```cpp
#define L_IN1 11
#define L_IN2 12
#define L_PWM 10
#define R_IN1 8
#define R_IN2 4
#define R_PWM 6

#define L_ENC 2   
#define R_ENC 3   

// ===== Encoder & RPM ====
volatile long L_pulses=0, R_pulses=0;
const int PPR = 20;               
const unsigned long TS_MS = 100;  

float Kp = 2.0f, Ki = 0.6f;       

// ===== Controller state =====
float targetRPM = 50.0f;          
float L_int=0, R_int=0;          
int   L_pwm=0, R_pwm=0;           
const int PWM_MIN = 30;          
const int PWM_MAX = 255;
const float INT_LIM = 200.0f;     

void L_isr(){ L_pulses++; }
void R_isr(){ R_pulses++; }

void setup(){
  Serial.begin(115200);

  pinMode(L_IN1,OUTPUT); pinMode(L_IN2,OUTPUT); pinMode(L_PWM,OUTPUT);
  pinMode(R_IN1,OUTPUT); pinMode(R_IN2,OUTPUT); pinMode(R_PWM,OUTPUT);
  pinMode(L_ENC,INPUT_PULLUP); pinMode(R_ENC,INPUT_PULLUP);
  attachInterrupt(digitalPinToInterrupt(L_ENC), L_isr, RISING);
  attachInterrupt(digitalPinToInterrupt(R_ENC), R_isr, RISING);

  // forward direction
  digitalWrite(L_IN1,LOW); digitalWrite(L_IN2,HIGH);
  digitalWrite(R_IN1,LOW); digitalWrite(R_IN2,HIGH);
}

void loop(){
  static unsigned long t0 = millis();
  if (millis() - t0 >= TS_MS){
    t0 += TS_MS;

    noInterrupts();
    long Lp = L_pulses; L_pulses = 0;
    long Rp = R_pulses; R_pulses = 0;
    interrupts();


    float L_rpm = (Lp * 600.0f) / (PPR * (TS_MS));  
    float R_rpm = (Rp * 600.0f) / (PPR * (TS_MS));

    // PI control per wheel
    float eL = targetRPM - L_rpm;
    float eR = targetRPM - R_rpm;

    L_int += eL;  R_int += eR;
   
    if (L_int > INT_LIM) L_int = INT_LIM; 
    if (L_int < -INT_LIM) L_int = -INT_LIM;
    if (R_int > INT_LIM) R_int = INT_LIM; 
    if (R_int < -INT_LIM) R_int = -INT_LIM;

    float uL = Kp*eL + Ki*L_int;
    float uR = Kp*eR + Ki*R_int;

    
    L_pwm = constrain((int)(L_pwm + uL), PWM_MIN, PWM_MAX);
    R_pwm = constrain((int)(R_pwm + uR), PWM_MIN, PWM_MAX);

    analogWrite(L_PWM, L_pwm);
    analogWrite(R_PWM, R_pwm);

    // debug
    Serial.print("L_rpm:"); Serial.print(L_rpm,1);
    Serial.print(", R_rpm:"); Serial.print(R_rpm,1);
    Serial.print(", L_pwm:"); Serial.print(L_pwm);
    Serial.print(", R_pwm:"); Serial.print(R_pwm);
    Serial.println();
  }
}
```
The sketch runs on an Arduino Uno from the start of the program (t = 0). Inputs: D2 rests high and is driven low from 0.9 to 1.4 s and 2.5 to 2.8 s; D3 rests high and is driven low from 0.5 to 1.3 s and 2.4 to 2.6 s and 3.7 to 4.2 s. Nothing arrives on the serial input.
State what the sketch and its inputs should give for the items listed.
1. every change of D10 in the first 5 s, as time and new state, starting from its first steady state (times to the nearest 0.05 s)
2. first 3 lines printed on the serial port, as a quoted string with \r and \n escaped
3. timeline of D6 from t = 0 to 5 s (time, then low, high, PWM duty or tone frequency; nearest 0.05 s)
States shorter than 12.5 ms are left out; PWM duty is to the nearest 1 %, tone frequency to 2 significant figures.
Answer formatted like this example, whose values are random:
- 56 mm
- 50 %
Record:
- 0 s low; 0.1 s PWM 51 %; 0.2 s high
- "L_rpm:0.0, R_rpm:0.0, L_pwm:130, R_pwm:130\r\nL_rpm:0.0, R_rpm:0.0, L_pwm:255, R_pwm:255\r\nL_rpm:0.0, R_rpm:0.0, L_pwm:255, R_pwm:255\r\n"
- 0 s low; 0.1 s PWM 51 %; 0.2 s high
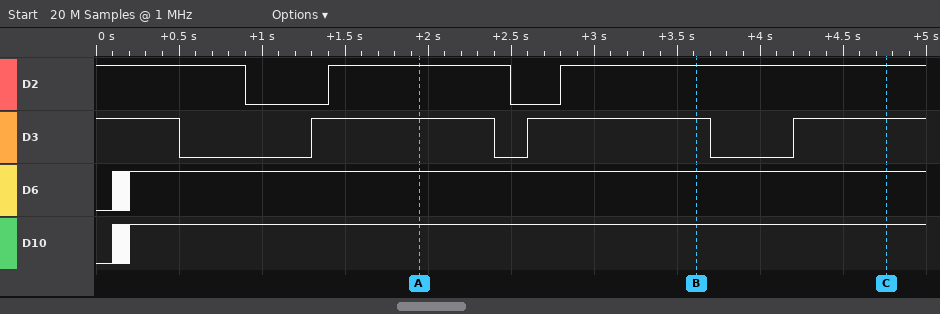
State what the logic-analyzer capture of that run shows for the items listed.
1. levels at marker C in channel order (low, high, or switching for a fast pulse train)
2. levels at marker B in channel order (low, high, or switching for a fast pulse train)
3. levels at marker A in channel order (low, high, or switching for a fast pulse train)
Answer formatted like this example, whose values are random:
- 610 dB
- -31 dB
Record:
- D2 high, D3 high, D6 high, D10 high
- D2 high, D3 high, D6 high, D10 high
- D2 high, D3 high, D6 high, D10 high
